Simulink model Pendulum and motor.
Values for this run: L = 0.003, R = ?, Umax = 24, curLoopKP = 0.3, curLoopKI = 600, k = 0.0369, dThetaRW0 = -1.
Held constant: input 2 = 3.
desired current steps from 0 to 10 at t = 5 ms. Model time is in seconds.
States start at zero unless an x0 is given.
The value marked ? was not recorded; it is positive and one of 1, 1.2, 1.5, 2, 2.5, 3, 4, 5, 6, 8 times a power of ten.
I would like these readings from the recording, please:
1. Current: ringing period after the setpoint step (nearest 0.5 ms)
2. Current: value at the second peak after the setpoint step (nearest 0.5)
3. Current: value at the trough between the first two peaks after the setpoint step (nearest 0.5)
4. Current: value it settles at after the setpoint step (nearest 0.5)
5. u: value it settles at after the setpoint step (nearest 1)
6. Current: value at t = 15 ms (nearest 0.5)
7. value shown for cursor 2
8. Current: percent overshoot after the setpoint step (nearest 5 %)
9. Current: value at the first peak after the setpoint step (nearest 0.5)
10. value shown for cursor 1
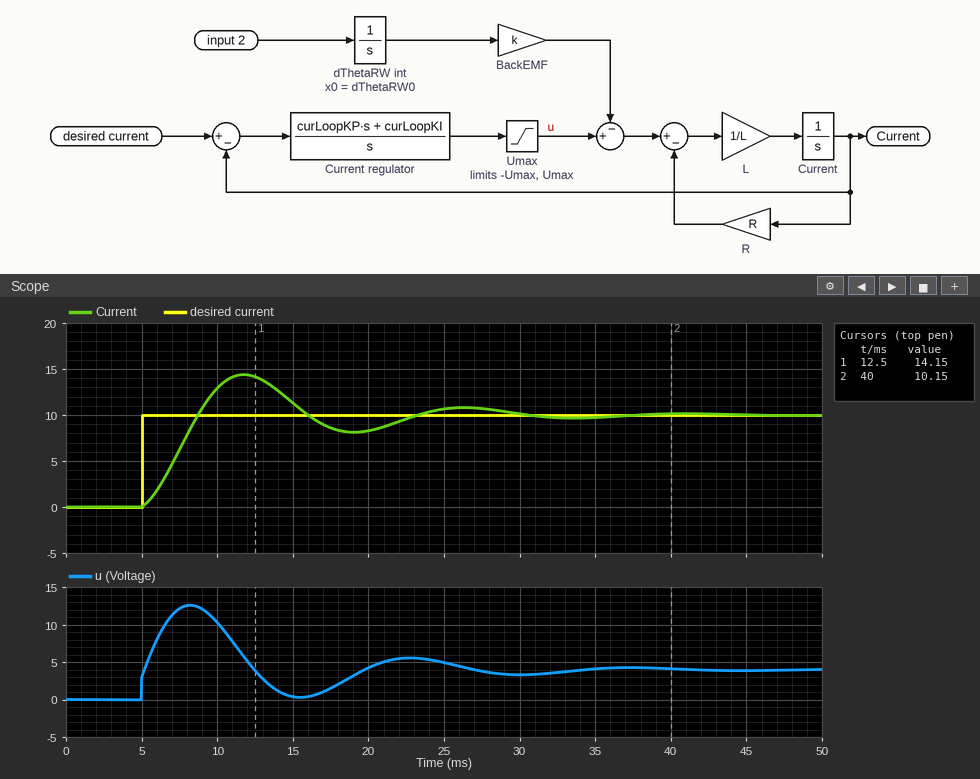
14.5 ms
11.0
8.0
10.0
4
11.5
10.15
45 %
14.5
14.15
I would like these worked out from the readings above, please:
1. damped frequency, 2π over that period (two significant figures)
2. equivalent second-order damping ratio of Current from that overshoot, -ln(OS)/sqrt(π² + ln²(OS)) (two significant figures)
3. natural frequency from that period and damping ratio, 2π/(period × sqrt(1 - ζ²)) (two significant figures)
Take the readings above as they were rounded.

0.43 rad/ms
0.25
0.45 rad/ms
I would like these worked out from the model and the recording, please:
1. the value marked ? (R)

0.4
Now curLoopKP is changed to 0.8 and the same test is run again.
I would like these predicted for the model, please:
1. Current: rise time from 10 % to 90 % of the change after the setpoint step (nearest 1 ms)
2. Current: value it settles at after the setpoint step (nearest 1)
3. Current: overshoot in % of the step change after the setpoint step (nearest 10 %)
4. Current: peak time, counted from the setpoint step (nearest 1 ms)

3 ms
10
30 %
6 ms
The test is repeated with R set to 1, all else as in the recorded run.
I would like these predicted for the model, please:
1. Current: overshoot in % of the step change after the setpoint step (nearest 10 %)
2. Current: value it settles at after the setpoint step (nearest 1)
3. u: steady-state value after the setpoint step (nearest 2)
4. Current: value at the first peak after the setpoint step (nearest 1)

20 %
10
10
12
